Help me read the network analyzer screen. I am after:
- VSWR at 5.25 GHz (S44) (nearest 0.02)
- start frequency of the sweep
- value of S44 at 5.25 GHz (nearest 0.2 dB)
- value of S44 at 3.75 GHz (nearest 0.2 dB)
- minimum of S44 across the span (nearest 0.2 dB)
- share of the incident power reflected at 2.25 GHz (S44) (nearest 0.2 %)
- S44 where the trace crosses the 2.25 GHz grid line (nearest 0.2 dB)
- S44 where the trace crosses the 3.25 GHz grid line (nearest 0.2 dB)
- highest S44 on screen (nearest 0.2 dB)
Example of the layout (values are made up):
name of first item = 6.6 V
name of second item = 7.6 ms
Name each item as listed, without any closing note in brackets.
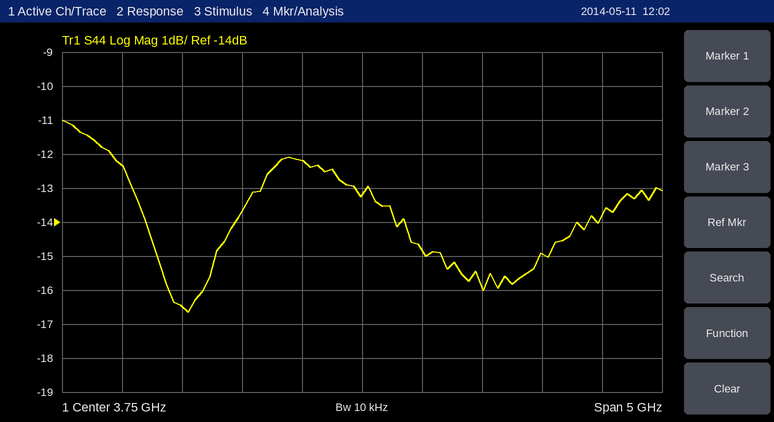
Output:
VSWR at 5.25 GHz (S44) = 1.44
start frequency of the sweep = 1.25 GHz
value of S44 at 5.25 GHz = -15.0 dB
value of S44 at 3.75 GHz = -13.2 dB
minimum of S44 across the span = -16.6 dB
share of the incident power reflected at 2.25 GHz (S44) = 2.2 %
S44 where the trace crosses the 2.25 GHz grid line = -16.4 dB
S44 where the trace crosses the 3.25 GHz grid line = -12.2 dB
highest S44 on screen = -11.0 dB
